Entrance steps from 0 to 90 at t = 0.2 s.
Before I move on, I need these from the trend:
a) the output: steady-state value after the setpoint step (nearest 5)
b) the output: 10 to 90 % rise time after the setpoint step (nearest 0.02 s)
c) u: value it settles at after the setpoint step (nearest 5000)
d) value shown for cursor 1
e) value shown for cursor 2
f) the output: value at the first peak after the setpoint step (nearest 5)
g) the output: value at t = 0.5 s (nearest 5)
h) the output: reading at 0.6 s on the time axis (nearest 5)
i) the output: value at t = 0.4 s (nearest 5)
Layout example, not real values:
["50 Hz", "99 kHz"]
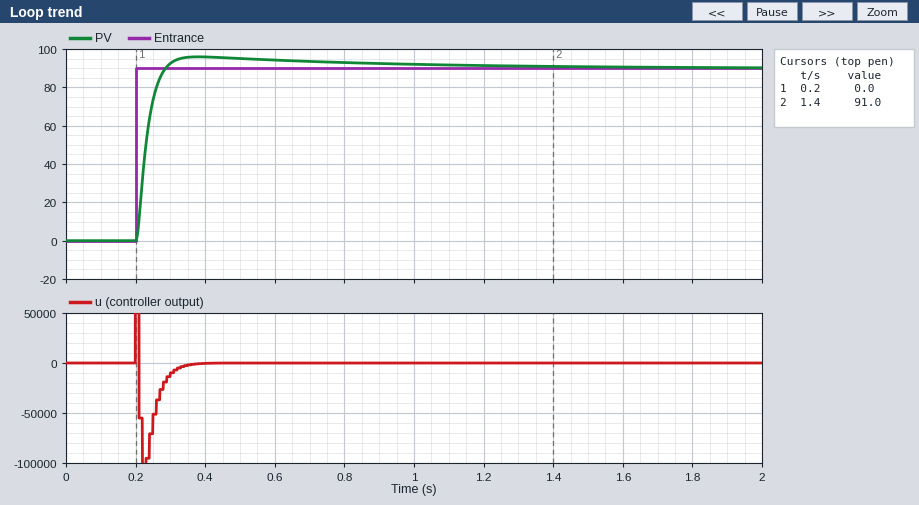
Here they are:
["90", "0.06 s", "0", "0.0", "91.0", "95", "95", "95", "95"]
